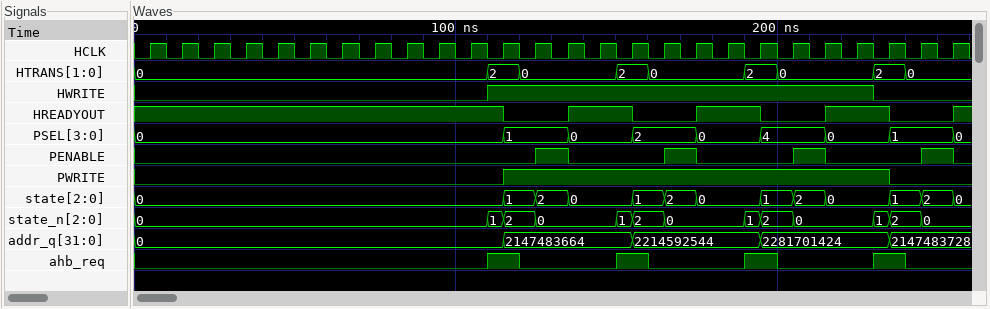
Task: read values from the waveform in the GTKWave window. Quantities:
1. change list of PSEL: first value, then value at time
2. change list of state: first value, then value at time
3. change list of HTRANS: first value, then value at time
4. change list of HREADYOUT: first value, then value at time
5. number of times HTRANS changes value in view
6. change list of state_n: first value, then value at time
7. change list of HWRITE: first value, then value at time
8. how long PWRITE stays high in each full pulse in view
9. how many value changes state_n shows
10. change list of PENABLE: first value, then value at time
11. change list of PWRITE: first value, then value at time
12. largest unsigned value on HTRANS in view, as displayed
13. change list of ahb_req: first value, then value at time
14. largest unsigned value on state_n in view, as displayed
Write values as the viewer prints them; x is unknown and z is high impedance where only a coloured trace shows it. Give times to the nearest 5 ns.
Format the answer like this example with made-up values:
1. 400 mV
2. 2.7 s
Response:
1. 0, 1 at 115 ns, 0 at 135 ns, 2 at 155 ns, 0 at 175 ns, 4 at 195 ns, 0 at 215 ns, 1 at 235 ns, 0 at 255 ns
2. 0, 1 at 115 ns, 2 at 125 ns, 0 at 135 ns, 1 at 155 ns, 2 at 165 ns, 0 at 175 ns, 1 at 195 ns, 2 at 205 ns, 0 at 215 ns, 1 at 235 ns, 2 at 245 ns, 0 at 255 ns
3. 0, 2 at 110 ns, 0 at 120 ns, 2 at 150 ns, 0 at 160 ns, 2 at 190 ns, 0 at 200 ns, 2 at 230 ns, 0 at 240 ns
4. 1, 0 at 115 ns, 1 at 135 ns, 0 at 155 ns, 1 at 175 ns, 0 at 195 ns, 1 at 215 ns, 0 at 235 ns, 1 at 255 ns
5. 8
6. 0, 1 at 110 ns, 2 at 115 ns, 0 at 125 ns, 1 at 150 ns, 2 at 155 ns, 0 at 165 ns, 1 at 190 ns, 2 at 195 ns, 0 at 205 ns, 1 at 230 ns, 2 at 235 ns, 0 at 245 ns
7. 0, 1 at 110 ns, 0 at 230 ns
8. 120 ns
9. 12
10. 0, 1 at 125 ns, 0 at 135 ns, 1 at 165 ns, 0 at 175 ns, 1 at 205 ns, 0 at 215 ns, 1 at 245 ns, 0 at 255 ns
11. 0, 1 at 115 ns, 0 at 235 ns
12. 2
13. 0, 1 at 110 ns, 0 at 120 ns, 1 at 150 ns, 0 at 160 ns, 1 at 190 ns, 0 at 200 ns, 1 at 230 ns, 0 at 240 ns
14. 2
